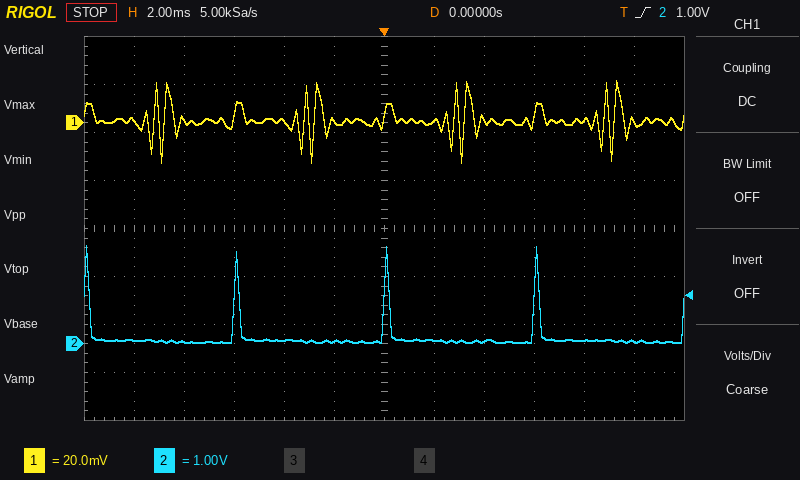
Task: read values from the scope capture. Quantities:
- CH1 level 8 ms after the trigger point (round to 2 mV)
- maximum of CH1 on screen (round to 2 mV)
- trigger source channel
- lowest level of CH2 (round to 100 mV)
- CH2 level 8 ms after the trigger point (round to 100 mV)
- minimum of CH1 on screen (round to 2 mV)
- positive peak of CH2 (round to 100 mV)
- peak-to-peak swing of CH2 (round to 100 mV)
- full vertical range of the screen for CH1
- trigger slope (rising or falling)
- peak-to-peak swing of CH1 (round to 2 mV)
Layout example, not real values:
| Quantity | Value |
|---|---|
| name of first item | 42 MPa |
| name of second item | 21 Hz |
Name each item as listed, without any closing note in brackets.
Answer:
| Quantity | Value |
|---|---|
| CH1 level 8 ms after the trigger point | 2 mV |
| maximum of CH1 on screen | 18 mV |
| trigger source channel | CH2 |
| lowest level of CH2 | 0.0 V |
| CH2 level 8 ms after the trigger point | 100 mV |
| minimum of CH1 on screen | -16 mV |
| positive peak of CH2 | 2.0 V |
| peak-to-peak swing of CH2 | 2.0 V |
| full vertical range of the screen for CH1 | 160 mV |
| trigger slope | rising |
| peak-to-peak swing of CH1 | 34 mV |
